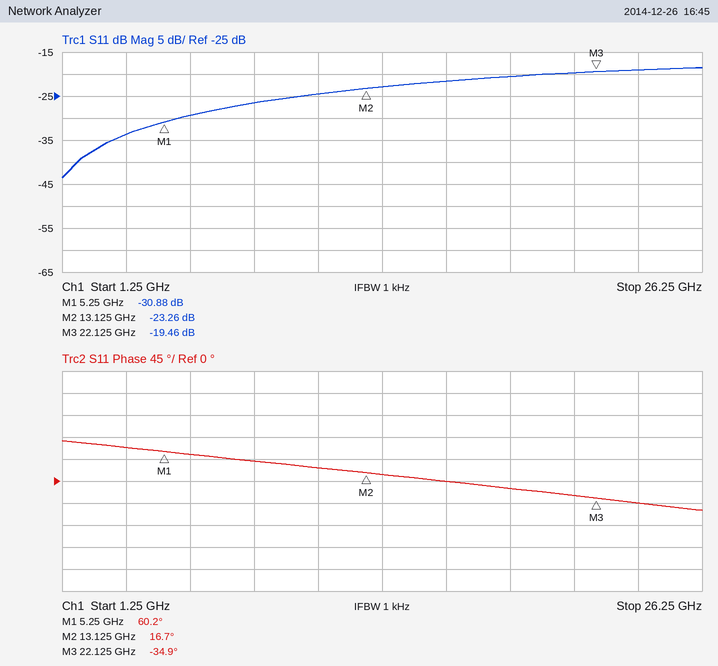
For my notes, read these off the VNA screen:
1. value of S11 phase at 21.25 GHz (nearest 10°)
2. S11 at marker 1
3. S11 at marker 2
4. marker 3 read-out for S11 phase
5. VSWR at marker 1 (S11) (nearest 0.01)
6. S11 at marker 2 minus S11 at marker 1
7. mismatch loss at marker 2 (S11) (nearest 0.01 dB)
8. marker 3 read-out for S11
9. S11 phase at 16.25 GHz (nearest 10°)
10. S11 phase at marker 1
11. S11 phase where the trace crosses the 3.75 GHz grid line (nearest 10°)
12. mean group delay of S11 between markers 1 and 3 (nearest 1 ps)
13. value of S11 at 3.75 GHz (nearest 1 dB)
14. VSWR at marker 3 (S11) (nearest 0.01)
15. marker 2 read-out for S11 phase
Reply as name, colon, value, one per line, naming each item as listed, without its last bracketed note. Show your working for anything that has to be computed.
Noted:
value of S11 phase at 21.25 GHz: -30°
S11 at marker 1: -30.88 dB
S11 at marker 2: -23.26 dB
marker 3 read-out for S11 phase: -34.9°
VSWR at marker 1 (S11): (1 + 0.0286)/(1 − 0.0286) ≈ 1.06
S11 at marker 2 minus S11 at marker 1: -23.26 − (-30.88) = 7.62 dB
mismatch loss at marker 2 (S11): −10 log10(1 − 10^(-23.26/10)) ≈ 0.02 dB
marker 3 read-out for S11: -19.46 dB
S11 phase at 16.25 GHz: 0°
S11 phase at marker 1: 60.2°
S11 phase where the trace crosses the 3.75 GHz grid line: 70°
mean group delay of S11 between markers 1 and 3: −(-34.9° − (60.2°))/(360° × 16.875 GHz) ≈ 16 ps
value of S11 at 3.75 GHz: -34 dB
VSWR at marker 3 (S11): (1 + 0.1064)/(1 − 0.1064) ≈ 1.24
marker 2 read-out for S11 phase: 16.7°
